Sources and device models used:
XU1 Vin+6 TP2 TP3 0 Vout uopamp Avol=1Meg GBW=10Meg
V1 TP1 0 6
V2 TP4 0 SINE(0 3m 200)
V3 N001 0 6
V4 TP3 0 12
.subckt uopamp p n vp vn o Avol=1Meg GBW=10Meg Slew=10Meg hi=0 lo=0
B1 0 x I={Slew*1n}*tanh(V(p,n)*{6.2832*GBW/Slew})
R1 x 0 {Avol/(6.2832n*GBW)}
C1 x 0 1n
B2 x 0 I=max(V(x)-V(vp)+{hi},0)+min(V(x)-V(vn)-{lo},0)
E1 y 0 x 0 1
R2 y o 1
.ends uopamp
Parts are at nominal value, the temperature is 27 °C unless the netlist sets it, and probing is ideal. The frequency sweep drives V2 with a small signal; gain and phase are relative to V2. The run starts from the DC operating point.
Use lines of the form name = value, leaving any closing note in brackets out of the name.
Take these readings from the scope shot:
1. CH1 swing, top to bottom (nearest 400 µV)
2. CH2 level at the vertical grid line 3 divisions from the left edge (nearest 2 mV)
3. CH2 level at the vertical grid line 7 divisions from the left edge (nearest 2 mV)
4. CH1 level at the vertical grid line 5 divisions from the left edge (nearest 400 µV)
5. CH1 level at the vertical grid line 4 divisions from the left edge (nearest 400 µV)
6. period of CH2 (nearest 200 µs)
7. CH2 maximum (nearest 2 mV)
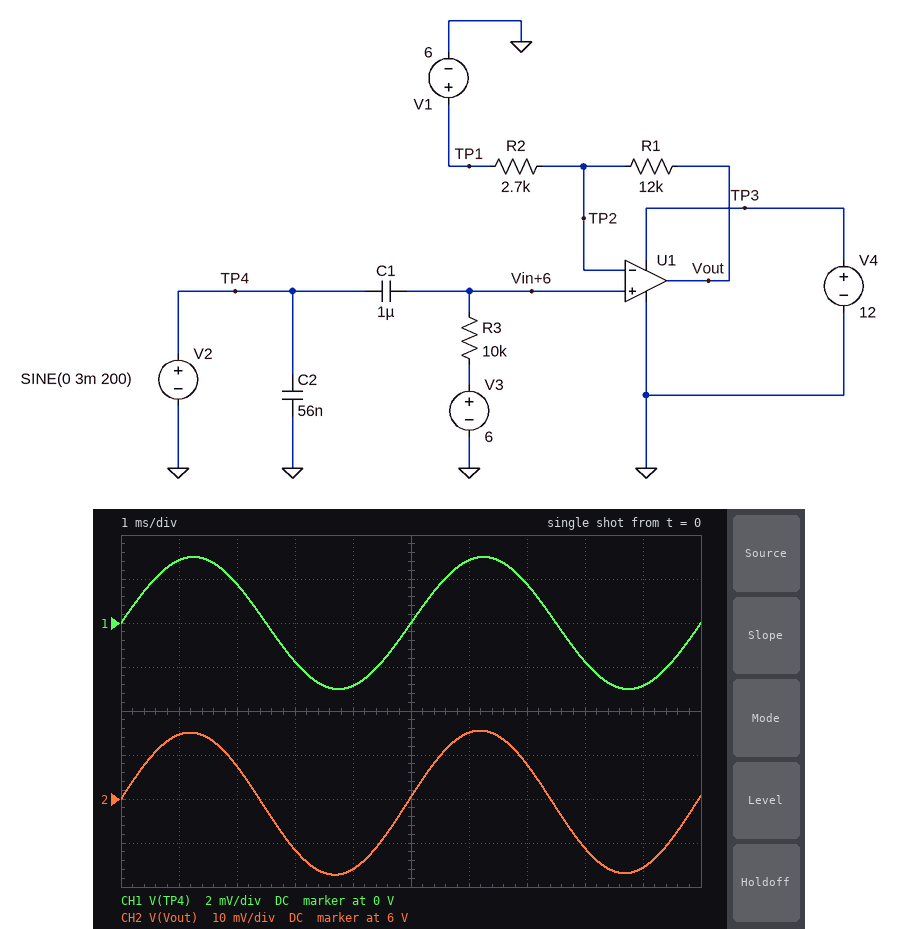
CH1 swing, top to bottom = 6.0 mV
CH2 level at the vertical grid line 3 divisions from the left edge = 5.988 V
CH2 level at the vertical grid line 7 divisions from the left edge = 6.008 V
CH1 level at the vertical grid line 5 divisions from the left edge = 0 V
CH1 level at the vertical grid line 4 divisions from the left edge = -2.8 mV
period of CH2 = 5.0 ms
CH2 maximum = 6.016 V
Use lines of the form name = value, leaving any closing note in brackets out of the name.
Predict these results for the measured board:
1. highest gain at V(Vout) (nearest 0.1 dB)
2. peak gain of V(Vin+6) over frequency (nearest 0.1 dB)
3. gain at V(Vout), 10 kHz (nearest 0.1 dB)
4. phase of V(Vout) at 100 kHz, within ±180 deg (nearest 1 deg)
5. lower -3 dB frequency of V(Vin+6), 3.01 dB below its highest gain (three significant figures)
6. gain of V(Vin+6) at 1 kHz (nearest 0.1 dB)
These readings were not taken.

highest gain at V(Vout) = 14.7 dB
peak gain of V(Vin+6) over frequency = 0 dB
gain at V(Vout), 10 kHz = 14.7 dB
phase of V(Vout) at 100 kHz, within ±180 deg = -3 deg
lower -3 dB frequency of V(Vin+6), 3.01 dB below its highest gain = 15.9 Hz
gain of V(Vin+6) at 1 kHz = 0 dB
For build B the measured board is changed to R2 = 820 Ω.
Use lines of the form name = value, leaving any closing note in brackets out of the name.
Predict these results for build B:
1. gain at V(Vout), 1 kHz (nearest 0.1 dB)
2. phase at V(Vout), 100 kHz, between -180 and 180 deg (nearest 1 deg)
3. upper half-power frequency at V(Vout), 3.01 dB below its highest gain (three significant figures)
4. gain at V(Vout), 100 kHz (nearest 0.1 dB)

gain at V(Vout), 1 kHz = 23.9 dB
phase at V(Vout), 100 kHz, between -180 and 180 deg = -9 deg
upper half-power frequency at V(Vout), 3.01 dB below its highest gain = 640 kHz
gain at V(Vout), 100 kHz = 23.8 dB
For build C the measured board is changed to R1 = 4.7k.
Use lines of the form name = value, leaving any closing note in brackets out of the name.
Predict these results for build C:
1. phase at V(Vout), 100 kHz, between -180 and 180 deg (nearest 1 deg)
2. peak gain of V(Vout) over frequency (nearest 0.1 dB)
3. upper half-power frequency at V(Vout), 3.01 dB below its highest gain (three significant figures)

phase at V(Vout), 100 kHz, between -180 and 180 deg = -2 deg
peak gain of V(Vout) over frequency = 8.8 dB
upper half-power frequency at V(Vout), 3.01 dB below its highest gain = 3.65 MHz
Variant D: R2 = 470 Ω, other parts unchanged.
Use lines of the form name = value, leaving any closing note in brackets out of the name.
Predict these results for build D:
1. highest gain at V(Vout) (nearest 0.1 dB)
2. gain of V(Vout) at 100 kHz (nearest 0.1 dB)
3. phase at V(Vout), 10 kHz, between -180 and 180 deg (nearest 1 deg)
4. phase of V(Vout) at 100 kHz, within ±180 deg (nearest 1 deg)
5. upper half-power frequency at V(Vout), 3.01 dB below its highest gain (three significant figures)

highest gain at V(Vout) = 28.5 dB
gain of V(Vout) at 100 kHz = 28.2 dB
phase at V(Vout), 10 kHz, between -180 and 180 deg = -1 deg
phase of V(Vout) at 100 kHz, within ±180 deg = -15 deg
upper half-power frequency at V(Vout), 3.01 dB below its highest gain = 377 kHz
